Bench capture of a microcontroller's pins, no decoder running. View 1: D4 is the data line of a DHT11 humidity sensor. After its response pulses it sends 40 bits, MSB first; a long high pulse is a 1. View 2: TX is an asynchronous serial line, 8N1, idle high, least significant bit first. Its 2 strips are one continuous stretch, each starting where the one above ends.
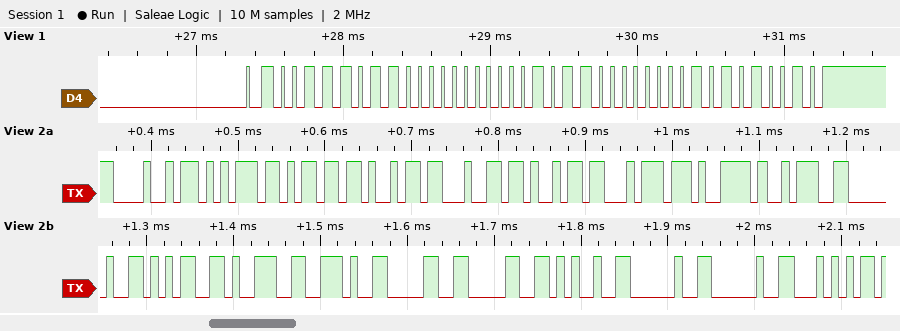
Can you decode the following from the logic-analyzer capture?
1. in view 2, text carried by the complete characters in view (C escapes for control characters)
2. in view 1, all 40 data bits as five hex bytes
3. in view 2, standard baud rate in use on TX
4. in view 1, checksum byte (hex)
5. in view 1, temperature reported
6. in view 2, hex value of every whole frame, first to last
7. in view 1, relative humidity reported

"Humidity: 59.00%  T"
3B 00 16 01 52
115200 baud
0x52
22.1 °C
48 75 6D 69 64 69 74 79 3A 20 35 39 2E 30 30 25 20 20 54
59 %
